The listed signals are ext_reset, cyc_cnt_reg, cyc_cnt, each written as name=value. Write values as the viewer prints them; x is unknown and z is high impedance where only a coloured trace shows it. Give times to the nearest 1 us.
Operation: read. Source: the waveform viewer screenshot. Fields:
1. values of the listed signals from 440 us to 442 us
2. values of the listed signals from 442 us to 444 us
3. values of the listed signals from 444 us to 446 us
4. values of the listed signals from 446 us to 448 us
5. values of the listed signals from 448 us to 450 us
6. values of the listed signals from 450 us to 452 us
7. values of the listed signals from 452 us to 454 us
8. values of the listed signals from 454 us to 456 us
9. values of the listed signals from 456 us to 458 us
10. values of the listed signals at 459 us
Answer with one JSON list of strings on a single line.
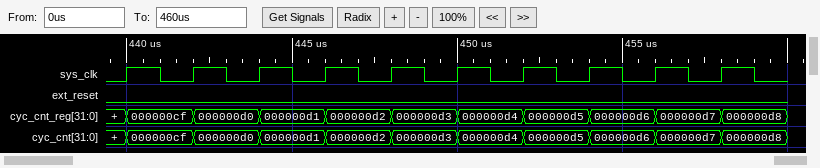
["ext_reset=0, cyc_cnt_reg=000000cf, cyc_cnt=000000cf", "ext_reset=0, cyc_cnt_reg=000000d0, cyc_cnt=000000d0", "ext_reset=0, cyc_cnt_reg=000000d1, cyc_cnt=000000d1", "ext_reset=0, cyc_cnt_reg=000000d2, cyc_cnt=000000d2", "ext_reset=0, cyc_cnt_reg=000000d3, cyc_cnt=000000d3", "ext_reset=0, cyc_cnt_reg=000000d4, cyc_cnt=000000d4", "ext_reset=0, cyc_cnt_reg=000000d5, cyc_cnt=000000d5", "ext_reset=0, cyc_cnt_reg=000000d6, cyc_cnt=000000d6", "ext_reset=0, cyc_cnt_reg=000000d7, cyc_cnt=000000d7", "ext_reset=0, cyc_cnt_reg=000000d8, cyc_cnt=000000d8"]
